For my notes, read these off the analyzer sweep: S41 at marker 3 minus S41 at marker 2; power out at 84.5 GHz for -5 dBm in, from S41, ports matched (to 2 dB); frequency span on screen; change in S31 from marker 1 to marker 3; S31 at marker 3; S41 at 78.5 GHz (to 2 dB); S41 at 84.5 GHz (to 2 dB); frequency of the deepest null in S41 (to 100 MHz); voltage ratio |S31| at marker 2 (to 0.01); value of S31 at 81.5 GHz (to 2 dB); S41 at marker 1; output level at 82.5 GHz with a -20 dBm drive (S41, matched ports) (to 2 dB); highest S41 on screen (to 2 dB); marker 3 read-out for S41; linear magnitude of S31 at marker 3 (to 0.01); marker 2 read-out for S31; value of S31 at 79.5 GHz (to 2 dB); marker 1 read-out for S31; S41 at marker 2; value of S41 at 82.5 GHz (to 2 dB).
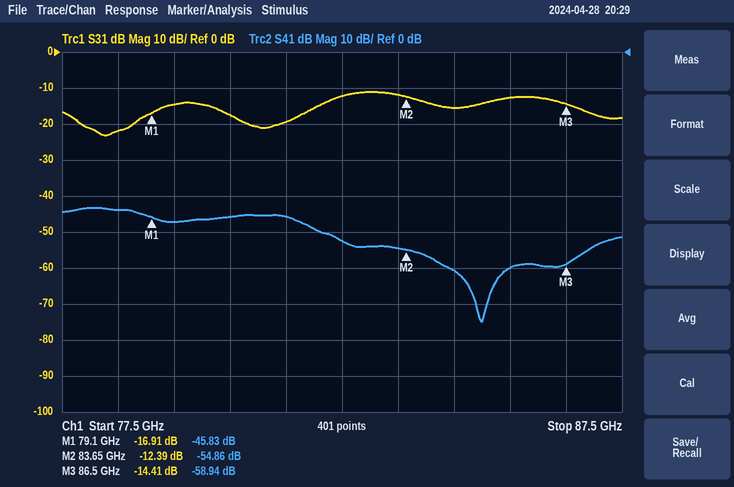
-4.08 dB
-66 dBm
10 GHz
2.50 dB
-14.41 dB
-44 dB
-60 dB
85.0 GHz
0.24
-20 dB
-45.83 dB
-72 dBm
-44 dB
-58.94 dB
0.19
-12.39 dB
-14 dB
-16.91 dB
-54.86 dB
-52 dB
